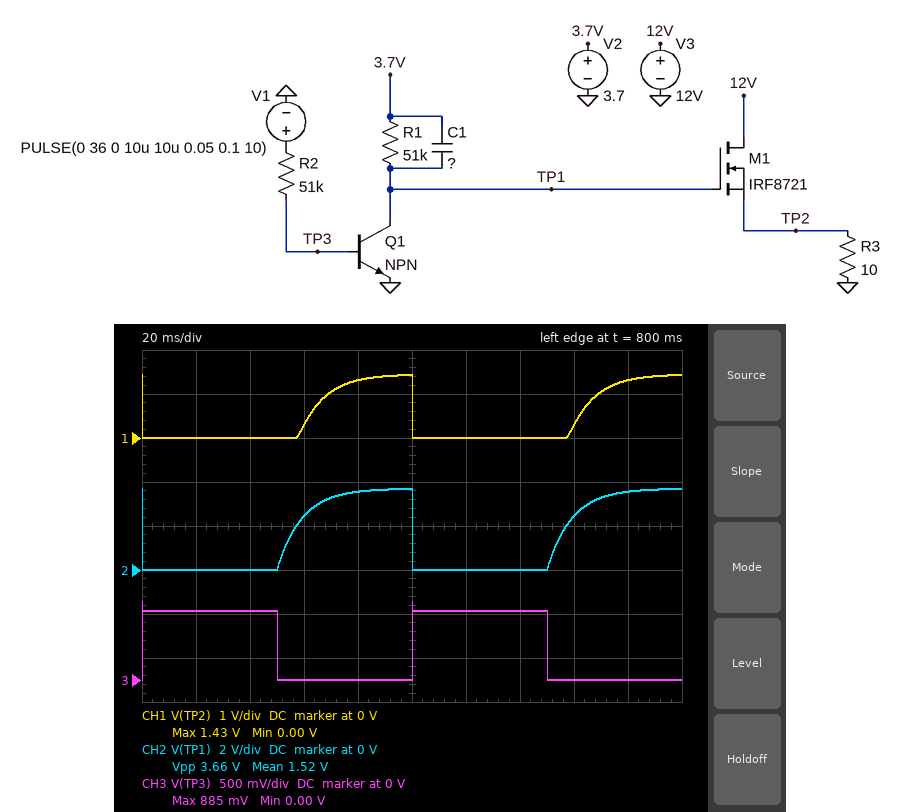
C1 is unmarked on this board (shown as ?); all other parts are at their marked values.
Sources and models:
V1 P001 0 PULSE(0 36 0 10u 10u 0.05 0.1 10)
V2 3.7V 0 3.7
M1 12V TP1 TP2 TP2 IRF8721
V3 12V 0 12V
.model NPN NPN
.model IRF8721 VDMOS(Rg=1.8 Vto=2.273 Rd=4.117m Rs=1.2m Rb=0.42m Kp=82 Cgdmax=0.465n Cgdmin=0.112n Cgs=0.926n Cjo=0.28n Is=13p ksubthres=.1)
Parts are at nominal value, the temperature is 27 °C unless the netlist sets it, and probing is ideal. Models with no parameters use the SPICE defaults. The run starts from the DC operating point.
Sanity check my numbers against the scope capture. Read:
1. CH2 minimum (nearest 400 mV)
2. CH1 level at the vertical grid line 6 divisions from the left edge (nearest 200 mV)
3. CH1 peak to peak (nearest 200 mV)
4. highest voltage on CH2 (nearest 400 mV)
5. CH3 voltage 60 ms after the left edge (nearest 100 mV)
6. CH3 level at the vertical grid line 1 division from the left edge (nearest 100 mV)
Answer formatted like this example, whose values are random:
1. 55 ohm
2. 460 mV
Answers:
1. 0 V
2. 0 V
3. 1.4 V
4. 3.6 V
5. 0 V
6. 800 mV
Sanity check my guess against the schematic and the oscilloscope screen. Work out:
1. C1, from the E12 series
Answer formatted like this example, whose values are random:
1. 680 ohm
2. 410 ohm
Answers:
1. 180 nF
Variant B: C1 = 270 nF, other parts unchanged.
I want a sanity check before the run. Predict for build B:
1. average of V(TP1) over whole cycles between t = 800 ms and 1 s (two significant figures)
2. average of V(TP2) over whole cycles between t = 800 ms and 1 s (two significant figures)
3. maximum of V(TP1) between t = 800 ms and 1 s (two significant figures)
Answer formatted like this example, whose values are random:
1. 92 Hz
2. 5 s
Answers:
1. 1.4 V
2. 360 mV
3. 3.6 V
